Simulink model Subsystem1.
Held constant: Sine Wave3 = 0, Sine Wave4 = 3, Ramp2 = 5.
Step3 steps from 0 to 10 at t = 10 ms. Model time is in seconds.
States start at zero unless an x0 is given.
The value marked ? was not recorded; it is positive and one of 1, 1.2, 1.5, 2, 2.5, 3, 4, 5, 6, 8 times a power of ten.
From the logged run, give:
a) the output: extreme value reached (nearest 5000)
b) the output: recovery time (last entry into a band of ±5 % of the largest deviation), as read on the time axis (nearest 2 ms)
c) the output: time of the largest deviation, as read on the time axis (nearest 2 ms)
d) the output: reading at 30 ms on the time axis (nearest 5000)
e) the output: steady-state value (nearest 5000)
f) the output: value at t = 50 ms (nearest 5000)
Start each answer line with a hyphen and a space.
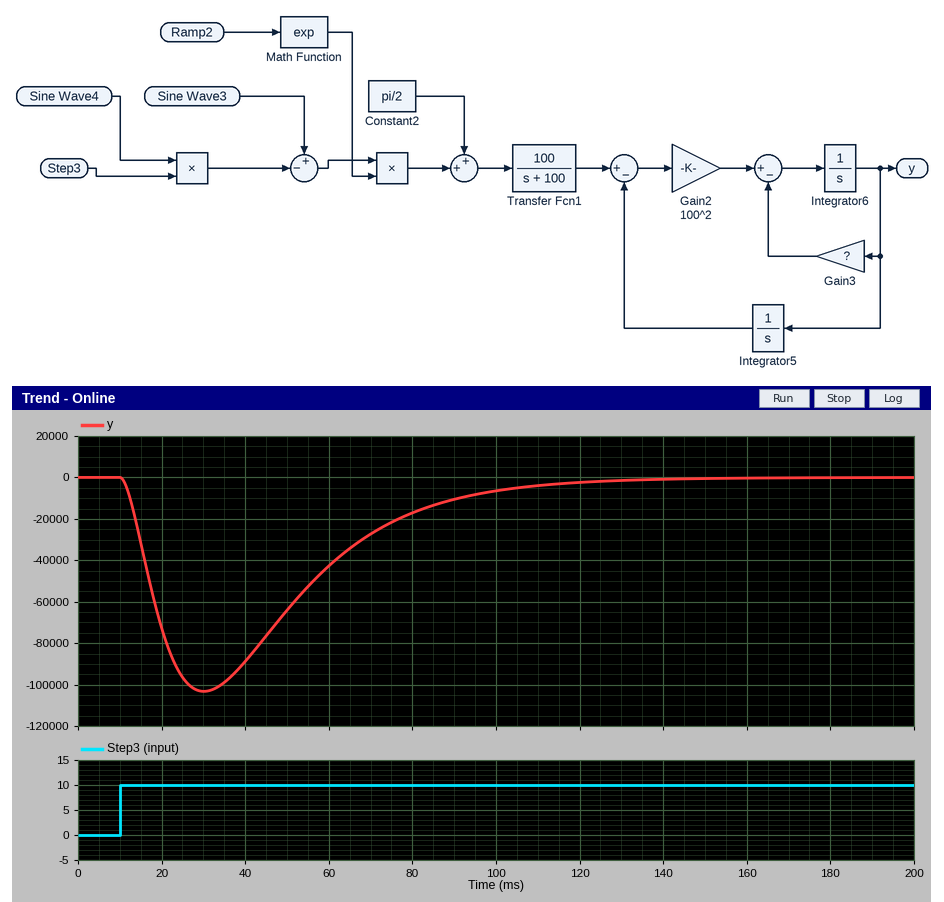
- -105000
- 104 ms
- 30 ms
- -105000
- 0
- -65000
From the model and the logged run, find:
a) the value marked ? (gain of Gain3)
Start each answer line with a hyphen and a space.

- 250
